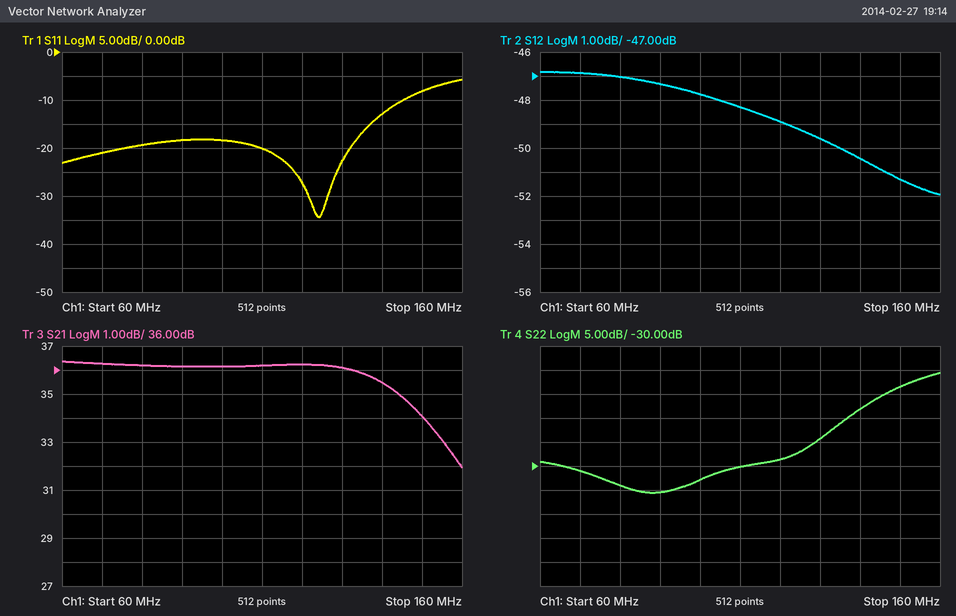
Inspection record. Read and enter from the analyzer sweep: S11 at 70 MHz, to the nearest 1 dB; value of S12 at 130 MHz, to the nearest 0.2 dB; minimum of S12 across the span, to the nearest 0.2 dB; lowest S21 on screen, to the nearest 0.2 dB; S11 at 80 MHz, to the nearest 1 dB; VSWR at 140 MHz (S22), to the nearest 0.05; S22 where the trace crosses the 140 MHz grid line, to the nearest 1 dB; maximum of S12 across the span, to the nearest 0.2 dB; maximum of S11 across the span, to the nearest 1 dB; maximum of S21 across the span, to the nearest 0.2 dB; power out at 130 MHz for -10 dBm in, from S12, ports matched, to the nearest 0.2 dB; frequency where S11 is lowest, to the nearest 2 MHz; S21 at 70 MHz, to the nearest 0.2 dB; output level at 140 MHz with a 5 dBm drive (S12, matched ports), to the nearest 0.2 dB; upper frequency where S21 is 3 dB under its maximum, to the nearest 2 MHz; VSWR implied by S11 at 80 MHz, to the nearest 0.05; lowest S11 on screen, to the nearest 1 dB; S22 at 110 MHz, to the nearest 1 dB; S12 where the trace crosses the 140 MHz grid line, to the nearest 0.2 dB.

-21 dB
-49.6 dB
-52.0 dB
32.0 dB
-19 dB
1.30
-18 dB
-46.8 dB
-6 dB
36.4 dB
-59.6 dBm
124 MHz
36.2 dB
-45.4 dBm
154 MHz
1.25
-34 dB
-30 dB
-50.4 dB
